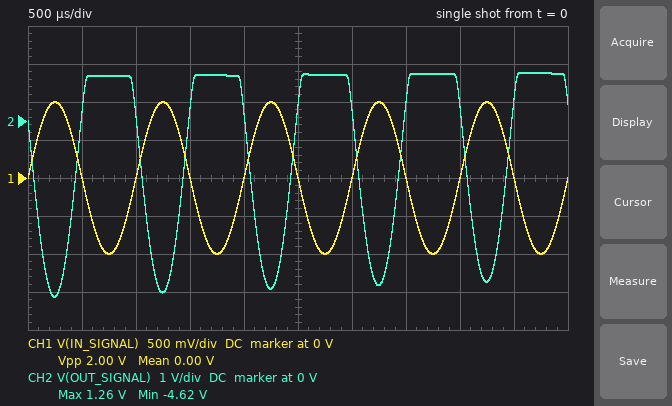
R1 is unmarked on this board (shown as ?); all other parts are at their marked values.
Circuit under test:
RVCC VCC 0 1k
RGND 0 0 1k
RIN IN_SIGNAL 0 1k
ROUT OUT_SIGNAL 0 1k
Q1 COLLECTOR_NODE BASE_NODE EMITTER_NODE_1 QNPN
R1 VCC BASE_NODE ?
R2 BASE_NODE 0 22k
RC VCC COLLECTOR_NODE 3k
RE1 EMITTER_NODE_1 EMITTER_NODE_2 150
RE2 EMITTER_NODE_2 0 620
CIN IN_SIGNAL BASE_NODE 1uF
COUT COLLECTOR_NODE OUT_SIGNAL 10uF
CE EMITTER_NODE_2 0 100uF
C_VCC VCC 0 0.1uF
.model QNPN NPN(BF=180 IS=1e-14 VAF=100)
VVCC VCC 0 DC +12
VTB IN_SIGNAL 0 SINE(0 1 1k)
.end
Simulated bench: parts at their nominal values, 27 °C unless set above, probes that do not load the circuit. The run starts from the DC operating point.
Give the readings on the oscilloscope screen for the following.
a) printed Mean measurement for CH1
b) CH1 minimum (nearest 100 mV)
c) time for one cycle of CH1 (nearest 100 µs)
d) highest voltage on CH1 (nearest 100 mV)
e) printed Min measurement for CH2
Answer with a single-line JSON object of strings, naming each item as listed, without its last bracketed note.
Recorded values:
{"printed Mean measurement for CH1": "0.00 V", "CH1 minimum": "-1.0 V", "time for one cycle of CH1": "1.0 ms", "highest voltage on CH1": "1.0 V", "printed Min measurement for CH2": "-4.62 V"}
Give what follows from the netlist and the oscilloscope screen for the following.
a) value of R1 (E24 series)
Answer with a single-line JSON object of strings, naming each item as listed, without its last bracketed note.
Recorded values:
{"value of R1": "110 kΩ"}
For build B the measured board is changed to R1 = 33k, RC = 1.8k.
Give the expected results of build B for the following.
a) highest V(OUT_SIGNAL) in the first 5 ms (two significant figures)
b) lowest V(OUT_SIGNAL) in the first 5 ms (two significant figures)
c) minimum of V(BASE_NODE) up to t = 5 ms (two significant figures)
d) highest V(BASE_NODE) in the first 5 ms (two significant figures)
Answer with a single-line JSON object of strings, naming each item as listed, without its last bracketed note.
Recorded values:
{"highest V(OUT_SIGNAL) in the first 5 ms": "2.9 V", "lowest V(OUT_SIGNAL) in the first 5 ms": "-720 mV", "minimum of V(BASE_NODE) up to t = 5 ms": "2.4 V", "highest V(BASE_NODE) in the first 5 ms": "4.7 V"}
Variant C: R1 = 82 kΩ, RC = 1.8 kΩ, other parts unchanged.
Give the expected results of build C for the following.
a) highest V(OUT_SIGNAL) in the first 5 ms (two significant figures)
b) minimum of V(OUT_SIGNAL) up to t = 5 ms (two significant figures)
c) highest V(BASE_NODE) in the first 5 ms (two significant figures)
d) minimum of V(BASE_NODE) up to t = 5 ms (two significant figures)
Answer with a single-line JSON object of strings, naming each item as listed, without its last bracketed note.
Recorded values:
{"highest V(OUT_SIGNAL) in the first 5 ms": "1.5 V", "minimum of V(OUT_SIGNAL) up to t = 5 ms": "-4.0 V", "highest V(BASE_NODE) in the first 5 ms": "3.3 V", "minimum of V(BASE_NODE) up to t = 5 ms": "1.3 V"}
